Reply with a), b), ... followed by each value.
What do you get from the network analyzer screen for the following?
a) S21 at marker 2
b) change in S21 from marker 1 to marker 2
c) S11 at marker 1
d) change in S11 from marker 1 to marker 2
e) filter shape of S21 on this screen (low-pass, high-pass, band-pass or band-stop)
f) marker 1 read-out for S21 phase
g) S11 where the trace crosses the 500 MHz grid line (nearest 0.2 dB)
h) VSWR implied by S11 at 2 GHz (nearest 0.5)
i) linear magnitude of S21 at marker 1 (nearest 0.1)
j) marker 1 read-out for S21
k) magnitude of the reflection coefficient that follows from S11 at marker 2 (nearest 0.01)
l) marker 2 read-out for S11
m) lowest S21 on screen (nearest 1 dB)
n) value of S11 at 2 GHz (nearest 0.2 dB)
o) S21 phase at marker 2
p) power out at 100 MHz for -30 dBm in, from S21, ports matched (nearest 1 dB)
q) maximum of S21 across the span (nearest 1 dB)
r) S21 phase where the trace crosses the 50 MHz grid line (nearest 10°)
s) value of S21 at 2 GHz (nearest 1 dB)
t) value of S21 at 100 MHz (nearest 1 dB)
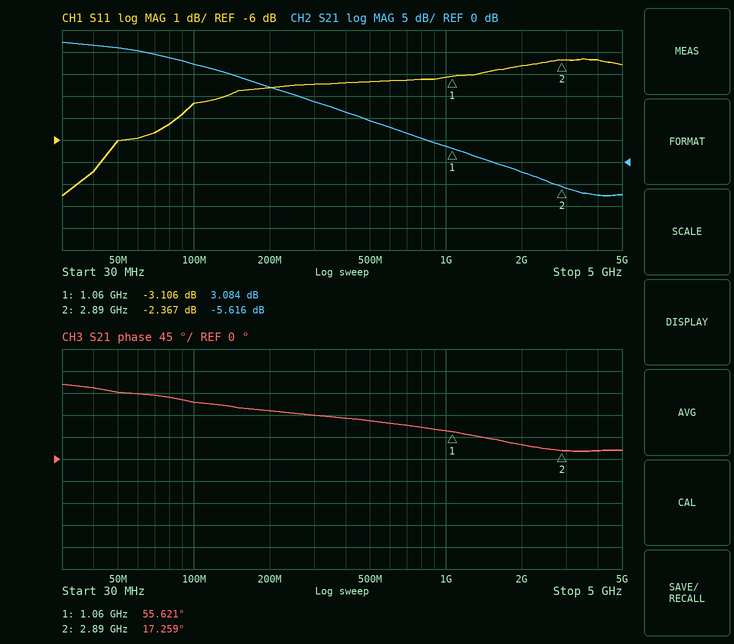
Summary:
a) -5.616 dB
b) -8.700 dB
c) -3.106 dB
d) 0.739 dB
e) low-pass
f) 55.621°
g) -3.4 dB
h) 6.5
i) 1.4
j) 3.084 dB
k) 0.76
l) -2.367 dB
m) -8 dB
n) -2.6 dB
o) 17.259°
p) -8 dBm
q) 27 dB
r) 140°
s) -2 dB
t) 22 dB
